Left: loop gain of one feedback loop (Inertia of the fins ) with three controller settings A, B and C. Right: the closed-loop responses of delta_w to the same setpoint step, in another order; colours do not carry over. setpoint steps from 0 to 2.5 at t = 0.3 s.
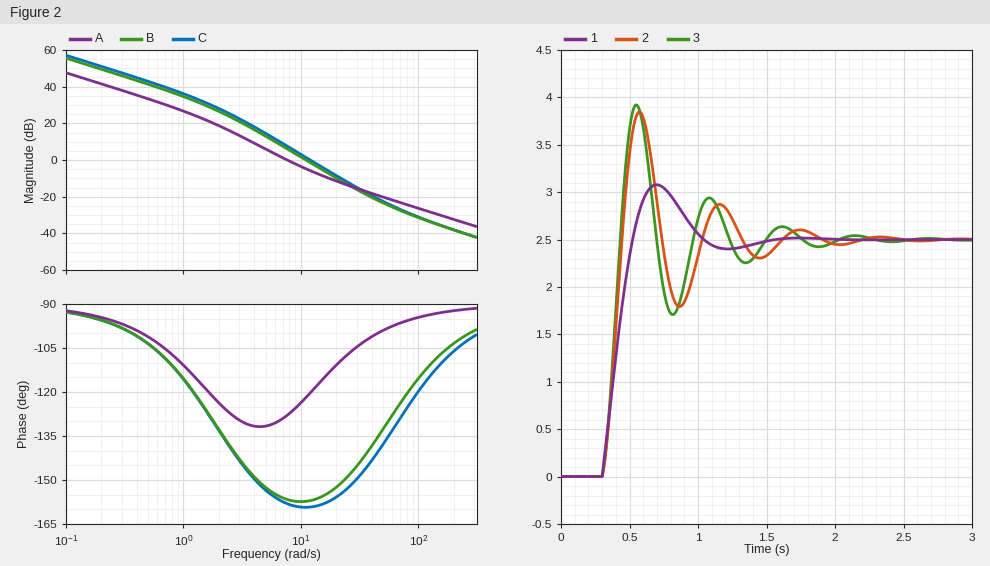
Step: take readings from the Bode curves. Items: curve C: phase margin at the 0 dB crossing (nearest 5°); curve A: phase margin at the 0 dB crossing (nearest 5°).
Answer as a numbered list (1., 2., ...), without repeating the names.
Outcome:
1. 20°
2. 50°
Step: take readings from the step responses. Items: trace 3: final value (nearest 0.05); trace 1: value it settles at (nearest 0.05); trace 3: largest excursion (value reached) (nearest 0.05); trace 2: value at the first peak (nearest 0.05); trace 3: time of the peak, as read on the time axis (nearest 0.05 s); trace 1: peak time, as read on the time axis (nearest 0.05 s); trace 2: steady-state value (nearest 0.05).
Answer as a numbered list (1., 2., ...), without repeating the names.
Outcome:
1. 2.50
2. 2.50
3. 3.90
4. 3.85
5. 0.55 s
6. 0.70 s
7. 2.50
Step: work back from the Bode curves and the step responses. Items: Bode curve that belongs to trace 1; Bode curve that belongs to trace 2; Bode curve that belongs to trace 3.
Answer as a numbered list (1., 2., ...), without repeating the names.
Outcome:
1. A
2. B
3. C
